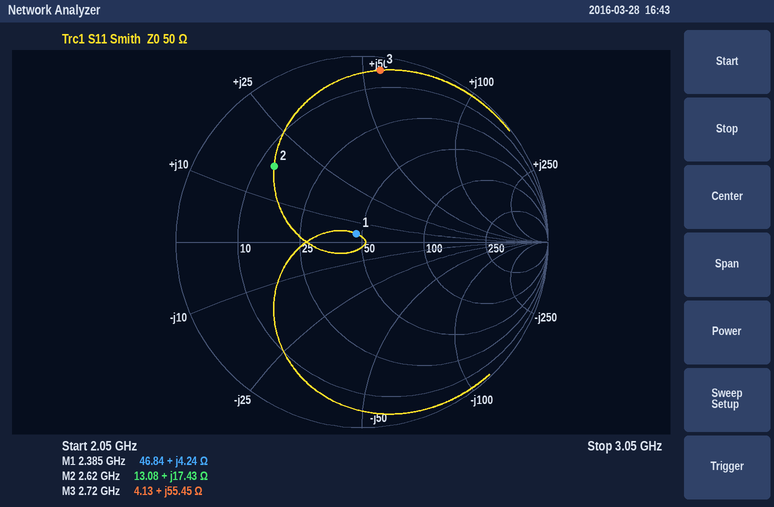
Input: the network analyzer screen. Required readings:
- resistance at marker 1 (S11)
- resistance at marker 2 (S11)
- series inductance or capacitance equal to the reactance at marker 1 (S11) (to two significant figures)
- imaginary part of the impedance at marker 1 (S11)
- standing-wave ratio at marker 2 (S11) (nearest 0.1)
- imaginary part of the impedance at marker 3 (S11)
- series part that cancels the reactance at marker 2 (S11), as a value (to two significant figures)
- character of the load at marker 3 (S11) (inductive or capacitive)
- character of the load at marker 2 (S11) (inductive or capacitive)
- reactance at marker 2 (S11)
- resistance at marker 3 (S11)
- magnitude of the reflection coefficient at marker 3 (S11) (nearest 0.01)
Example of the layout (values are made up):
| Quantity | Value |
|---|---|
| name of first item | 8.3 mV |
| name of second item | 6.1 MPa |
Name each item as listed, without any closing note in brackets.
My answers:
| Quantity | Value |
|---|---|
| resistance at marker 1 | 46.84 Ω |
| resistance at marker 2 | 13.08 Ω |
| series inductance or capacitance equal to the reactance at marker 1 (S11) | 280 pH |
| imaginary part of the impedance at marker 1 | +4.24 Ω |
| standing-wave ratio at marker 2 (S11) | 4.3 |
| imaginary part of the impedance at marker 3 | +55.45 Ω |
| series part that cancels the reactance at marker 2 (S11), as a value | 3.5 pF |
| character of the load at marker 3 (S11) | inductive |
| character of the load at marker 2 (S11) | inductive |
| reactance at marker 2 | +17.43 Ω |
| resistance at marker 3 | 4.13 Ω |
| magnitude of the reflection coefficient at marker 3 (S11) | 0.93 |
